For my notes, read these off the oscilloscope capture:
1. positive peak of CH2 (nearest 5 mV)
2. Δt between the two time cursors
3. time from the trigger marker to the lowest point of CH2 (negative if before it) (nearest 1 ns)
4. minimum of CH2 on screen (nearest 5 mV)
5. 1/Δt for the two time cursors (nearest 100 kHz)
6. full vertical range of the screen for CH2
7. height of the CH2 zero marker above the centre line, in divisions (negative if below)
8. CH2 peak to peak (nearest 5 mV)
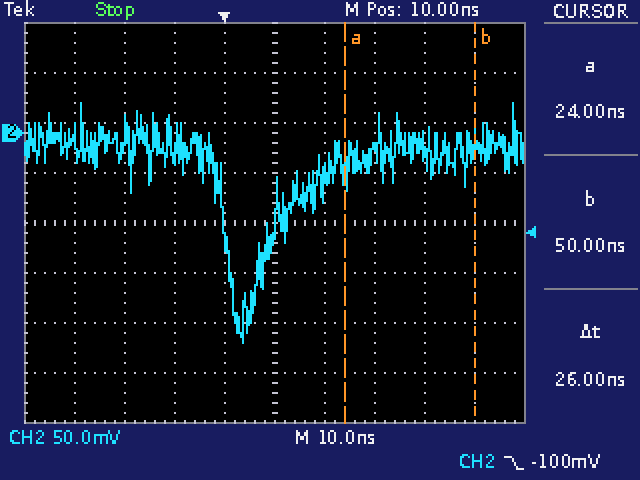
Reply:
30 mV
26 ns
+4 ns
-210 mV
38.5 MHz
400 mV
+1.8 div
240 mV
